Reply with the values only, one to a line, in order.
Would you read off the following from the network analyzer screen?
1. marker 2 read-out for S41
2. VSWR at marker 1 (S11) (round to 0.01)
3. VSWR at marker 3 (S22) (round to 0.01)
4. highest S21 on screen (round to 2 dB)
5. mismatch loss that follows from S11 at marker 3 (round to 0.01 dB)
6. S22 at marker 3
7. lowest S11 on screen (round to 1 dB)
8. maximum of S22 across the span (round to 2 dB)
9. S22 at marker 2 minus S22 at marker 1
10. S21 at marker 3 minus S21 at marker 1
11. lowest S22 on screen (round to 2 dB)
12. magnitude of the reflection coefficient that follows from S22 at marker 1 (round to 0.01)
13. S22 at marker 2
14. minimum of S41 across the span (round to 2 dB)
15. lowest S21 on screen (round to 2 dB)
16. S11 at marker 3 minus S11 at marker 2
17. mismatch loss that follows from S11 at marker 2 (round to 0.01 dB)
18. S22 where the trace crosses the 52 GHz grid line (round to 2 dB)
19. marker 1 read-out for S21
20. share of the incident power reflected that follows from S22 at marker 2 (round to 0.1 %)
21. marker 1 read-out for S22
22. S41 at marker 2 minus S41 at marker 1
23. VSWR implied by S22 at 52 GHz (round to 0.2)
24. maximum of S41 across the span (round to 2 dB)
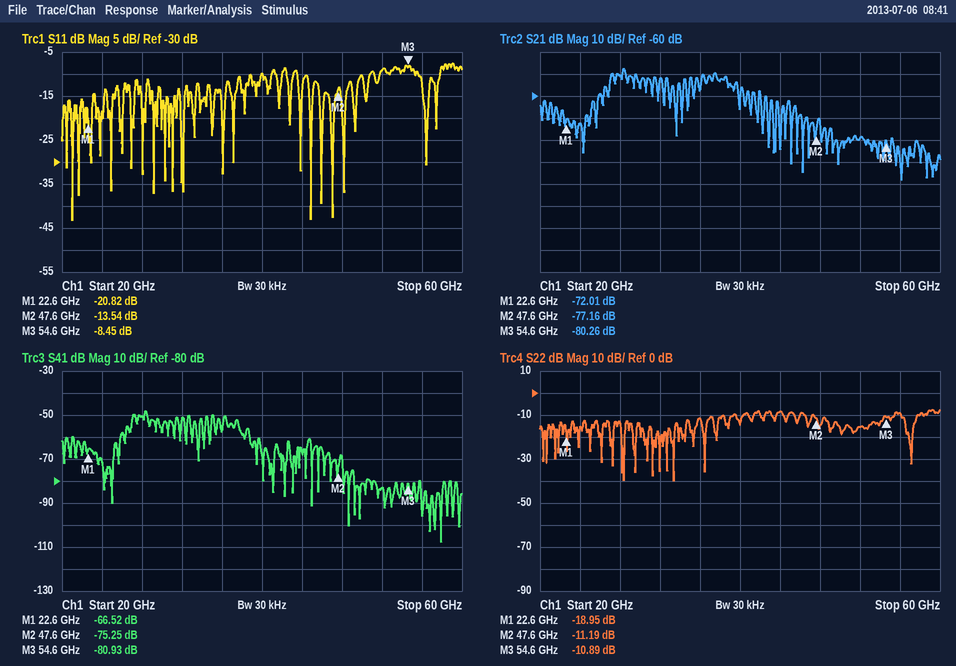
-75.25 dB
1.20
1.80
-48 dB
0.67 dB
-10.89 dB
-43 dB
-8 dB
7.76 dB
-8.25 dB
-40 dB
0.11
-11.19 dB
-108 dB
-98 dB
5.09 dB
0.20 dB
-16 dB
-72.01 dB
7.6 %
-18.95 dB
-8.73 dB
1.4
-48 dB
